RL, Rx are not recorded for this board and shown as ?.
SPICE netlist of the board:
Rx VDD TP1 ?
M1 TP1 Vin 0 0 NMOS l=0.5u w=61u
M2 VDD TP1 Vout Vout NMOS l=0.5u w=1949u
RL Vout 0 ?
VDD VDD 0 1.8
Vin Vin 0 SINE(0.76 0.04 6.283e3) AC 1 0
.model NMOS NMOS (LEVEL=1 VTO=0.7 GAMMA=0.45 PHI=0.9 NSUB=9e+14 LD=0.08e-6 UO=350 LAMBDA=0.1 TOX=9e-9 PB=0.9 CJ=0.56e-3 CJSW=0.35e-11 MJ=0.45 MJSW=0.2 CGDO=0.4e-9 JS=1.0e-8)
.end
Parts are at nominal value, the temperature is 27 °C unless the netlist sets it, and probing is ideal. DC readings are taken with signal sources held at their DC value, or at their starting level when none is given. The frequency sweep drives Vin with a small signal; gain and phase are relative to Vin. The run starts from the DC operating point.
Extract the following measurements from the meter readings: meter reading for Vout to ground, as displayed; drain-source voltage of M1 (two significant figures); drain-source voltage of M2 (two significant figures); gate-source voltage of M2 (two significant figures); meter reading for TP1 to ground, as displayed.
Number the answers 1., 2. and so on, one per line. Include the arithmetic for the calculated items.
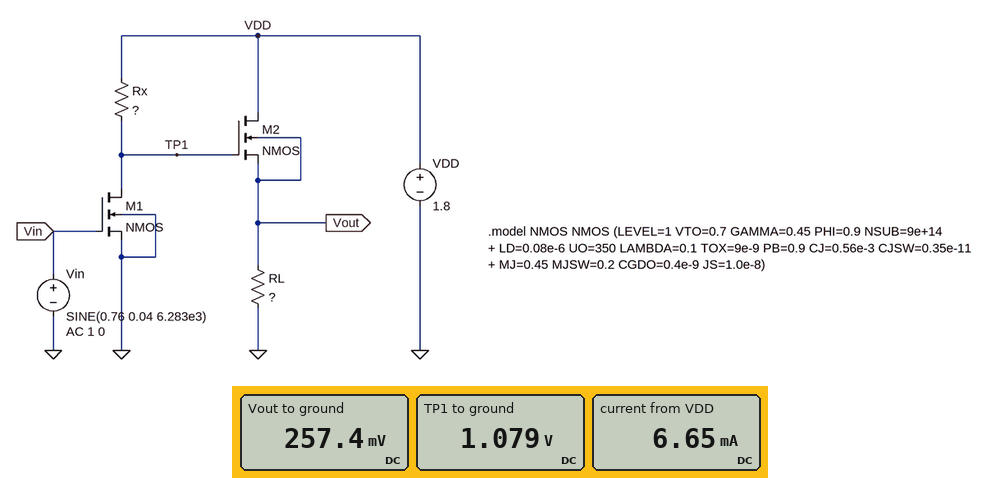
1. 257.4 mV
2. 1.079 V = 1.1 V
3. 1.8 V - 257.4 mV = 1.5 V
4. 1.079 V - 257.4 mV = 820 mV
5. 1.079 V
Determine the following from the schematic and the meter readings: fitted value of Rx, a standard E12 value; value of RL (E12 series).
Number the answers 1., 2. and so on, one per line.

1. 15 kΩ
2. 39 Ω
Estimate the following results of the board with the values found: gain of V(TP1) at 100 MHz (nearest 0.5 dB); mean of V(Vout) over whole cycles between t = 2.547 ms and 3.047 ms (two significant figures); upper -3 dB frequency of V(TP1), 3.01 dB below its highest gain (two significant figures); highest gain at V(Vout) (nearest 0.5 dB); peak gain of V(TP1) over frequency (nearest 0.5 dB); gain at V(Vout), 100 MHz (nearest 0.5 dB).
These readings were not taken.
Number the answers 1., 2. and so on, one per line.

1. 7.0 dB
2. 330 mV
3. 10 MHz
4. 25.0 dB
5. 27.0 dB
6. 5.0 dB
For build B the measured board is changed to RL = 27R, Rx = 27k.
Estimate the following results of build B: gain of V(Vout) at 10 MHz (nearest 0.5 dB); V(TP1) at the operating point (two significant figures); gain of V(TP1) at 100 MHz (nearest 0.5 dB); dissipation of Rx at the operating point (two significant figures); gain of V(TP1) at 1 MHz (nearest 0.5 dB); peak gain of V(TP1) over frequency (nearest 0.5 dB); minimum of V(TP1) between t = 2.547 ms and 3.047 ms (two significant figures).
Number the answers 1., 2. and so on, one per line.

1. -31.5 dB
2. 560 mV
3. 0 dB
4. 57 µW
5. 31.0 dB
6. 31.5 dB
7. 32 mV
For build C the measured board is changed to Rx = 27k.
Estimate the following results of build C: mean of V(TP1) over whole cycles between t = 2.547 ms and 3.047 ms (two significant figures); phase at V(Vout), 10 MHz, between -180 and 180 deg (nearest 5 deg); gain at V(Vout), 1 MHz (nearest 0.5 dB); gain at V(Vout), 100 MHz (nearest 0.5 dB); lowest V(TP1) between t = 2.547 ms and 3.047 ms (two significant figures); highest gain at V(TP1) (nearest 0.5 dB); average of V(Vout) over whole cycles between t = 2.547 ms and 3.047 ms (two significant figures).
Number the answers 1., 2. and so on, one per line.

1. 710 mV
2. -165 deg
3. -37.5 dB
4. -28.0 dB
5. 32 mV
6. 31.5 dB
7. 230 mV
